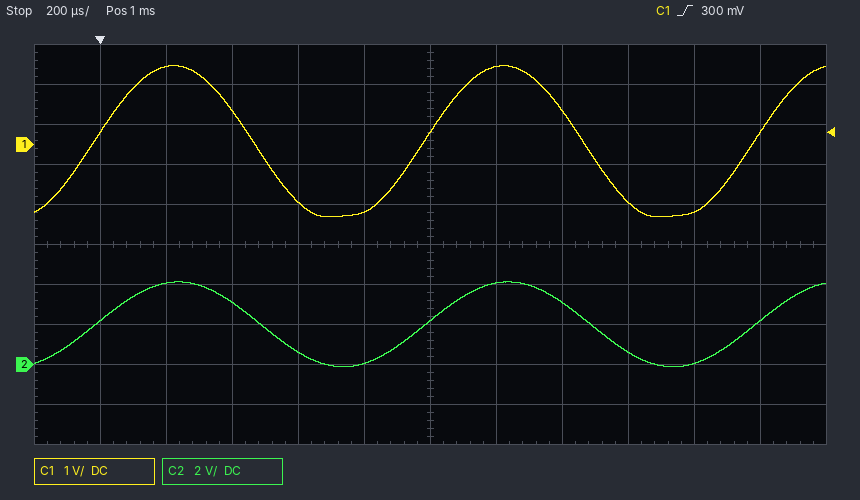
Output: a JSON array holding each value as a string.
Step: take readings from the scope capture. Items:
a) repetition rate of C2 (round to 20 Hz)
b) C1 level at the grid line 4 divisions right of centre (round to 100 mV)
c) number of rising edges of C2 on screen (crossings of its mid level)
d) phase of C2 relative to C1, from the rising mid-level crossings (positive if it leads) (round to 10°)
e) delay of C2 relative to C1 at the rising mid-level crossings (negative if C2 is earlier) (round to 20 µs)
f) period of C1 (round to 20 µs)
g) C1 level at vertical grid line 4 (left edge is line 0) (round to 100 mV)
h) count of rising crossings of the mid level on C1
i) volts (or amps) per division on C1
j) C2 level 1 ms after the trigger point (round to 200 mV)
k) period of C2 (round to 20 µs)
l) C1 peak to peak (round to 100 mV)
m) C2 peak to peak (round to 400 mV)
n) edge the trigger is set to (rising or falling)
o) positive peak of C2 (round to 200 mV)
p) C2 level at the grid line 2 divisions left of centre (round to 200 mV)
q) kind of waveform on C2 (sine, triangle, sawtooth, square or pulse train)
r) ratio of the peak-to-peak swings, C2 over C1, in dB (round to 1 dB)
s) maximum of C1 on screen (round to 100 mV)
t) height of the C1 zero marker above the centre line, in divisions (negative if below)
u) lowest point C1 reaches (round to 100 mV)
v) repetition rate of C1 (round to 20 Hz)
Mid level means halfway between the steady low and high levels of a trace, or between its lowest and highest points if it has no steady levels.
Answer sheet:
["1.00 kHz", "-1.7 V", "3", "0°", "0 µs", "1.00 ms", "-1.4 V", "3", "1 V", "2.2 V", "1.00 ms", "3.8 V", "4.4 V", "rising", "4.2 V", "600 mV", "sine", "1 dB", "2.0 V", "+2.5 div", "-1.8 V", "1.00 kHz"]
